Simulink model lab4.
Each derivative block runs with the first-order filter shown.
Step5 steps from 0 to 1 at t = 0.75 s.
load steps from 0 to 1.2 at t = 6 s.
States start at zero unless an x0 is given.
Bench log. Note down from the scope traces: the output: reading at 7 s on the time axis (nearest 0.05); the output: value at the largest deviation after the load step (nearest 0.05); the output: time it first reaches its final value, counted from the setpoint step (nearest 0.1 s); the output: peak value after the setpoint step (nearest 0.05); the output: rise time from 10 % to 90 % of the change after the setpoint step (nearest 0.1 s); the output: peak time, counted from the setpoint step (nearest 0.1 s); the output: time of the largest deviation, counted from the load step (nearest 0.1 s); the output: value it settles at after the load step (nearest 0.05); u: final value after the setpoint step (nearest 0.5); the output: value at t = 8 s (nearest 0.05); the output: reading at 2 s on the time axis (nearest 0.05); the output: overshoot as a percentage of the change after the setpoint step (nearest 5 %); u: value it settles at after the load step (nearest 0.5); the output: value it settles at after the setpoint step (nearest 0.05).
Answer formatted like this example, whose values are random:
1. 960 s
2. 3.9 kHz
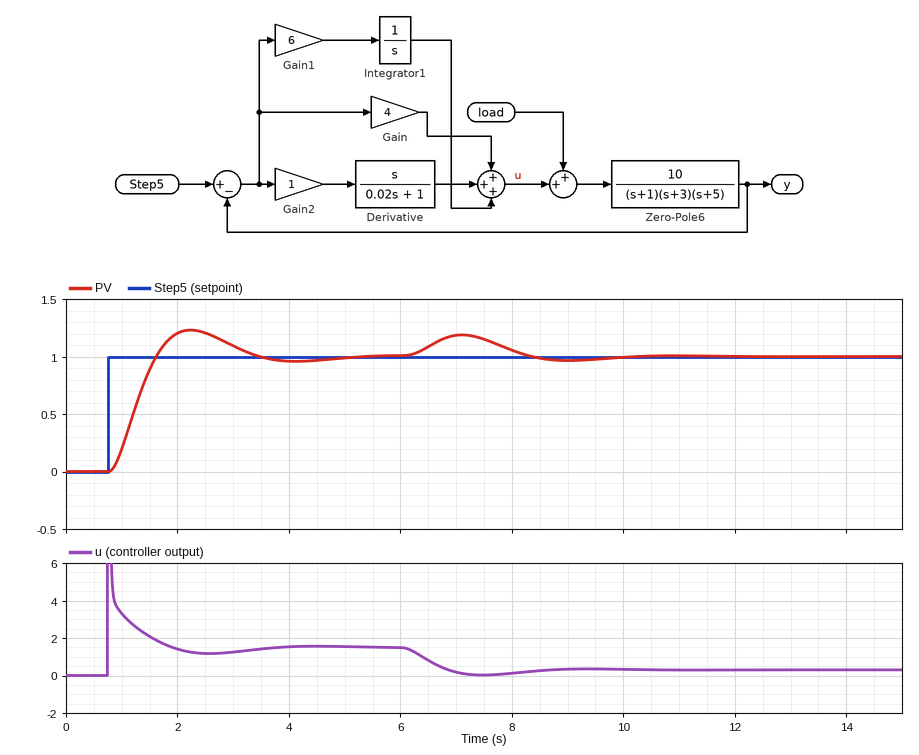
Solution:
1. 1.20
2. 1.20
3. 0.9 s
4. 1.25
5. 0.6 s
6. 1.5 s
7. 1.1 s
8. 1.00
9. 1.5
10. 1.05
11. 1.20
12. 25 %
13. 0.5
14. 1.00
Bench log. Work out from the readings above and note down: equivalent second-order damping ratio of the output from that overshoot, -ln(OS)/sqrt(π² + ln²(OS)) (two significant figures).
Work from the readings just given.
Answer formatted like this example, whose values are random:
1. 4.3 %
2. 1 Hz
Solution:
1. 0.40
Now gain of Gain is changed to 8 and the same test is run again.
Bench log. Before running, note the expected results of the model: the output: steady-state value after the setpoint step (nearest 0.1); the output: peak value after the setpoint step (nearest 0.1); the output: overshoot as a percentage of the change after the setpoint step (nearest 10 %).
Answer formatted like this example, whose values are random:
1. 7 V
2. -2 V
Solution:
1. 1.0
2. 1.3
3. 30 %
